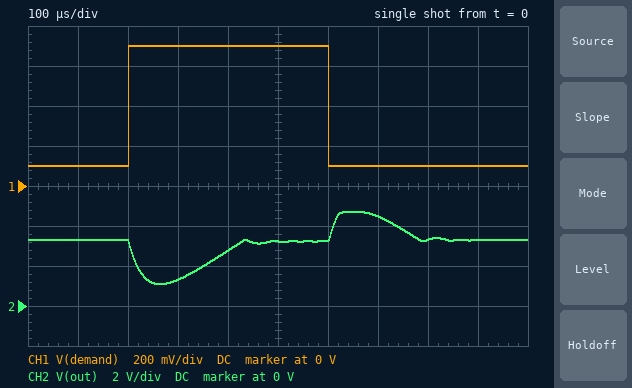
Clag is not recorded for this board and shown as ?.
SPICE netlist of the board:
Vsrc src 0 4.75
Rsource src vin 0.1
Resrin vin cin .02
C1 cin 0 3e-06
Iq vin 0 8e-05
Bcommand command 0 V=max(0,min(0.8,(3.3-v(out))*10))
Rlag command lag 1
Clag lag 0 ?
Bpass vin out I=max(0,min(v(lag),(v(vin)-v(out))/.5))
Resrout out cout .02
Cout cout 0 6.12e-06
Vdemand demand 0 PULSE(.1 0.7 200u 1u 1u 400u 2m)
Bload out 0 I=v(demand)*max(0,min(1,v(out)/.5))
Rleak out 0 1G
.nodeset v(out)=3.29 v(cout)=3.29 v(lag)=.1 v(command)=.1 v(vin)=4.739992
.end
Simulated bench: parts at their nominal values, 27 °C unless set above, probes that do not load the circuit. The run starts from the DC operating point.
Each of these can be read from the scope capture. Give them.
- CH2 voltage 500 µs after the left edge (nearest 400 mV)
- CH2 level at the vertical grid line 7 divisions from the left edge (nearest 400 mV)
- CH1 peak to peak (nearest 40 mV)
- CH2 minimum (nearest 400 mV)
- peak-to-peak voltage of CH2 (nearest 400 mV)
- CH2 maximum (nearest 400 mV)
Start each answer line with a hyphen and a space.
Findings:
- 3.2 V
- 4.4 V
- 600 mV
- 1.2 V
- 3.6 V
- 4.8 V
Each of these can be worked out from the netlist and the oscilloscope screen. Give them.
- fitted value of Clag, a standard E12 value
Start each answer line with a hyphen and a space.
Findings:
- 33 µF
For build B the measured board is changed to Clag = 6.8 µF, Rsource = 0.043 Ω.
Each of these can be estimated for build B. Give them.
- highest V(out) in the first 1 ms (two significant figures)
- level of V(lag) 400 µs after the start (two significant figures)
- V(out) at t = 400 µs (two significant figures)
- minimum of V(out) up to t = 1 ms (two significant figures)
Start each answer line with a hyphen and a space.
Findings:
- 3.7 V
- 700 mV
- 3.2 V
- 2.8 V
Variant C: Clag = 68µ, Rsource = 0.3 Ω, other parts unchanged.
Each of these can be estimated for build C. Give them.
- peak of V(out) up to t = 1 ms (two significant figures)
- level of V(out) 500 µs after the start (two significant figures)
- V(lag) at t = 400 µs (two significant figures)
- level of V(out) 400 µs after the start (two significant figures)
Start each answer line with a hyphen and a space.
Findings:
- 4.7 V
- 2.2 V
- 760 mV
- 900 mV
